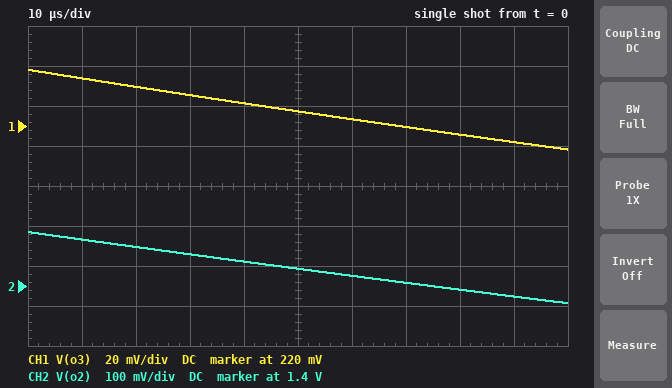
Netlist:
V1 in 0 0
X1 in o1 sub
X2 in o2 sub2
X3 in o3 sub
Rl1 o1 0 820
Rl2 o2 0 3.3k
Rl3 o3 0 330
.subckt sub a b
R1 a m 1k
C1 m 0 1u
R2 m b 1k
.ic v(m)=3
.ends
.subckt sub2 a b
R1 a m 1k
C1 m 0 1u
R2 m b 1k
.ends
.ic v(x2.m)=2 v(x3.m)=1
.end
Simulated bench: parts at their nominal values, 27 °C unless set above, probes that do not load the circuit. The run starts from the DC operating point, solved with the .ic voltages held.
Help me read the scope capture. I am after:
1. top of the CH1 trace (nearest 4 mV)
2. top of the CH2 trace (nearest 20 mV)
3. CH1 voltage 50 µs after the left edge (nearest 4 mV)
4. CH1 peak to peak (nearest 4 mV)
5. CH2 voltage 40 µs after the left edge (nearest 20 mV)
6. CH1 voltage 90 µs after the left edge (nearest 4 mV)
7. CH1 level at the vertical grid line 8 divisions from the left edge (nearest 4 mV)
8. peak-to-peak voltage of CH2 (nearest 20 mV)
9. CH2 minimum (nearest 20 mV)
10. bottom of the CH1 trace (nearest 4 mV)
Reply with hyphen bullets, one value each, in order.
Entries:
- 248 mV
- 1.54 V
- 228 mV
- 40 mV
- 1.46 V
- 212 mV
- 216 mV
- 180 mV
- 1.36 V
- 208 mV
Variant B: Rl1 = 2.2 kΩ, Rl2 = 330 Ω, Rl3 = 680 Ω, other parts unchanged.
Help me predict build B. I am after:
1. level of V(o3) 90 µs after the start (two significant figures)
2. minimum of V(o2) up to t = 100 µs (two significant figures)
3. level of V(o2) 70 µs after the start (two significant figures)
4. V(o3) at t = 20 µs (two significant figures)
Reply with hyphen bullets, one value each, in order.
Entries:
- 350 mV
- 420 mV
- 440 mV
- 390 mV
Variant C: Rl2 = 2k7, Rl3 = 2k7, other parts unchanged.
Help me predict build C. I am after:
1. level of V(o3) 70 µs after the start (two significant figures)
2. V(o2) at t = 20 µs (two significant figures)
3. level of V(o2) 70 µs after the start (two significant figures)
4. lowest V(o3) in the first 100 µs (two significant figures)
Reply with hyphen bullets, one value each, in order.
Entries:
- 670 mV
- 1.4 V
- 1.3 V
- 640 mV
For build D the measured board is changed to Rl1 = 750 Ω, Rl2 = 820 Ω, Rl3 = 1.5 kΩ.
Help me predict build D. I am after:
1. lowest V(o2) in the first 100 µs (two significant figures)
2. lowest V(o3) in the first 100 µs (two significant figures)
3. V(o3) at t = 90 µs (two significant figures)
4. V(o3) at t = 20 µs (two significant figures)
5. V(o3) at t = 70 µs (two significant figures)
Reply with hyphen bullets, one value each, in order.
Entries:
- 770 mV
- 520 mV
- 530 mV
- 580 mV
- 540 mV
